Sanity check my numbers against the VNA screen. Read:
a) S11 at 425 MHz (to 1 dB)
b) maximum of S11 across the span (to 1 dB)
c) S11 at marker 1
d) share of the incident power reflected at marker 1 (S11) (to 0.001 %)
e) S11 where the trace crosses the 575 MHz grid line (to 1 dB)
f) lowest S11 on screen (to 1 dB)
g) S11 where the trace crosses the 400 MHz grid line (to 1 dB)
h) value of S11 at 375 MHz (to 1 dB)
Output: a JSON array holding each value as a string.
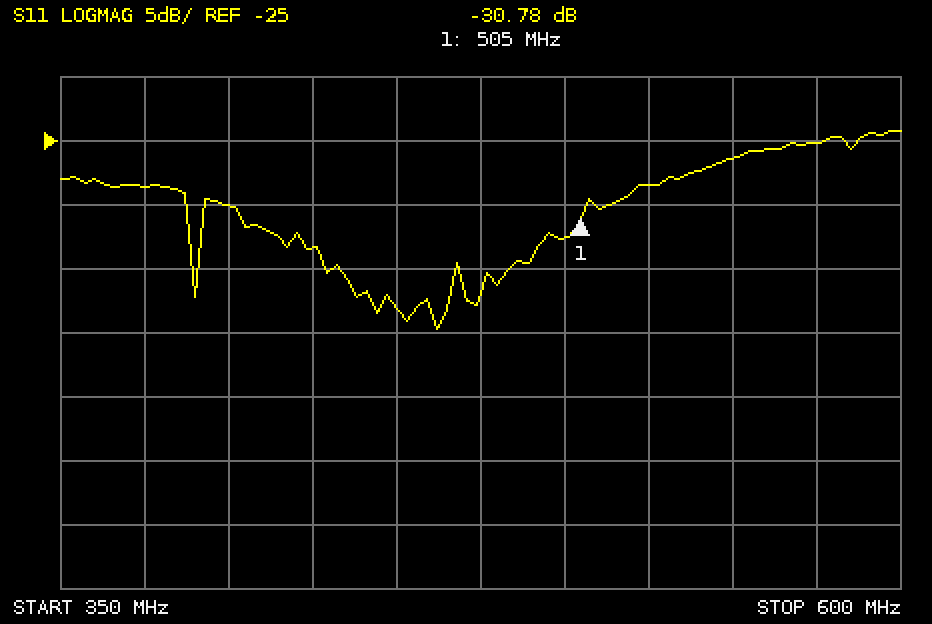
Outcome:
["-33 dB", "-24 dB", "-30.78 dB", "0.084 %", "-25 dB", "-40 dB", "-30 dB", "-29 dB"]
